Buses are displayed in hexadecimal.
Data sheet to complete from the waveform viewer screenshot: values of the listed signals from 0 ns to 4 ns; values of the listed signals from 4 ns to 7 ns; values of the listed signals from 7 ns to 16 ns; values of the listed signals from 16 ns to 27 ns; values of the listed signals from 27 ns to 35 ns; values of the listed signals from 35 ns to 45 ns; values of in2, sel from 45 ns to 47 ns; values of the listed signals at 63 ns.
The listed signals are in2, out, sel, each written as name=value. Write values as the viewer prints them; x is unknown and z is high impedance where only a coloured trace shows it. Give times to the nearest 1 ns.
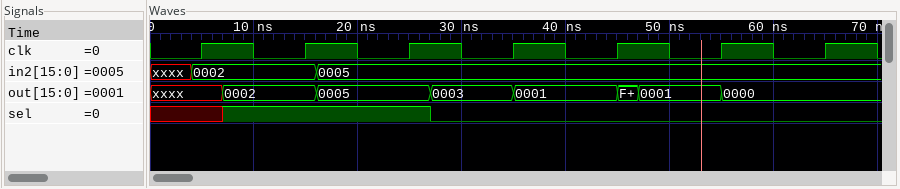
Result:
in2=xxxx, out=xxxx, sel=x
in2=0002, out=xxxx, sel=x
in2=0002, out=0002, sel=1
in2=0005, out=0005, sel=1
in2=0005, out=0003, sel=0
in2=0005, out=0001, sel=0
in2=0005, sel=0
in2=0005, out=0000, sel=0
